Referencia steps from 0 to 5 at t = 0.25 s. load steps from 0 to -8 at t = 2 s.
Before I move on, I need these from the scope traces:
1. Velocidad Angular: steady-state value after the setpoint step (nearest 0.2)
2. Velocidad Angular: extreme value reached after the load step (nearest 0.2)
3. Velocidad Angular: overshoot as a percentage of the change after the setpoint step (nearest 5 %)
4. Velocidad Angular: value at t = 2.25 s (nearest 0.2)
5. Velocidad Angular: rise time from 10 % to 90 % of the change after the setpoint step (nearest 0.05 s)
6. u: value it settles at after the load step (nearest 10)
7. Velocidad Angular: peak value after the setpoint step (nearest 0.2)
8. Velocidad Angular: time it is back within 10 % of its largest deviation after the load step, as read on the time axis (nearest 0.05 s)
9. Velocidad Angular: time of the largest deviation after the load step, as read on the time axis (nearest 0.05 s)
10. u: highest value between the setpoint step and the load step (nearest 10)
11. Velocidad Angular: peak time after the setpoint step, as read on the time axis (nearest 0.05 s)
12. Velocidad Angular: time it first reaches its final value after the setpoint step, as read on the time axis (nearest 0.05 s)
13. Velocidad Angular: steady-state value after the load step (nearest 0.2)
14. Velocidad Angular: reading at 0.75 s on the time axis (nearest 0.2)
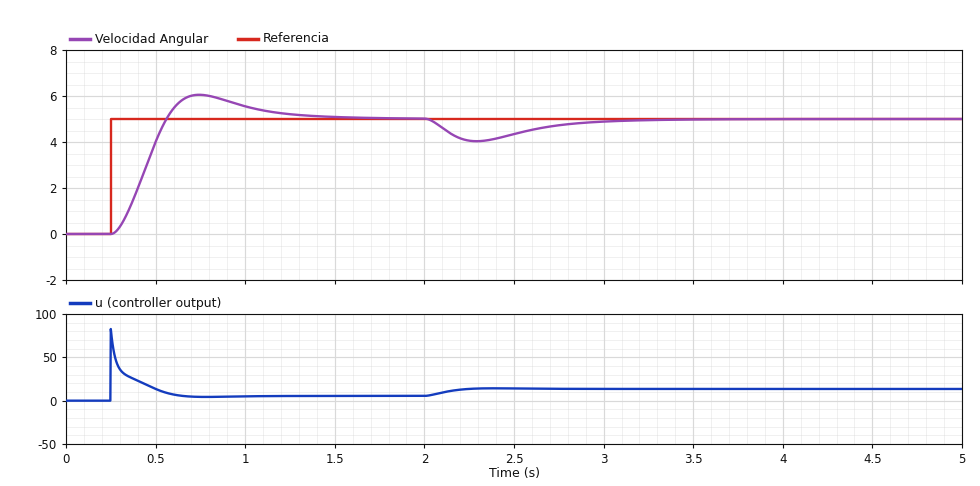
5.0
4.0
20 %
4.0
0.20 s
10
6.0
3.05 s
2.30 s
80
0.75 s
0.55 s
5.0
6.0
